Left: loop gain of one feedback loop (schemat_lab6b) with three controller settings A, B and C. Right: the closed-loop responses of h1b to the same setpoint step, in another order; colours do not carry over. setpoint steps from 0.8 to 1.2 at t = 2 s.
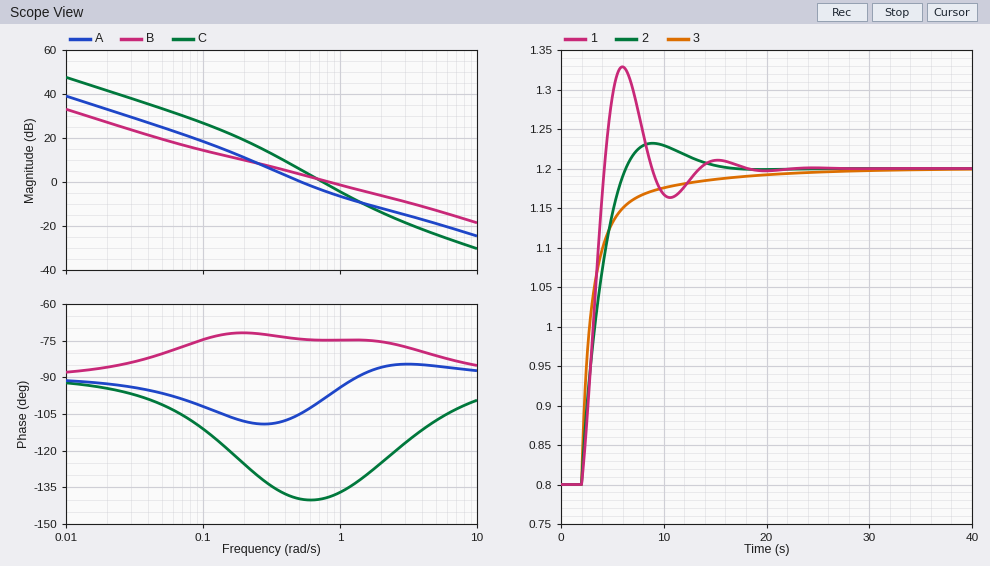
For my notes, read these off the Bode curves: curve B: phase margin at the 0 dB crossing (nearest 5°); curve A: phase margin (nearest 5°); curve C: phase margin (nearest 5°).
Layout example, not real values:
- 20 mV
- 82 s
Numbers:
- 105°
- 75°
- 40°
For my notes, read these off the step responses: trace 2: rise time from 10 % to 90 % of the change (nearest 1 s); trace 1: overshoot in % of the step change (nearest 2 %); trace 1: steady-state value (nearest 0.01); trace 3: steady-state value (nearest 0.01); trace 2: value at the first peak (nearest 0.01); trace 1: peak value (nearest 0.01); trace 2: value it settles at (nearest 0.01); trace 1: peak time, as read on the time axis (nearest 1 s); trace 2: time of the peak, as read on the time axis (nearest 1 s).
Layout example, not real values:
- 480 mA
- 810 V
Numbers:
- 3 s
- 32 %
- 1.20
- 1.20
- 1.23
- 1.33
- 1.20
- 6 s
- 9 s
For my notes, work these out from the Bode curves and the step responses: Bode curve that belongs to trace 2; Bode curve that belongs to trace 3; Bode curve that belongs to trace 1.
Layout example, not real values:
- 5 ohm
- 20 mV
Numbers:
- A
- B
- C
